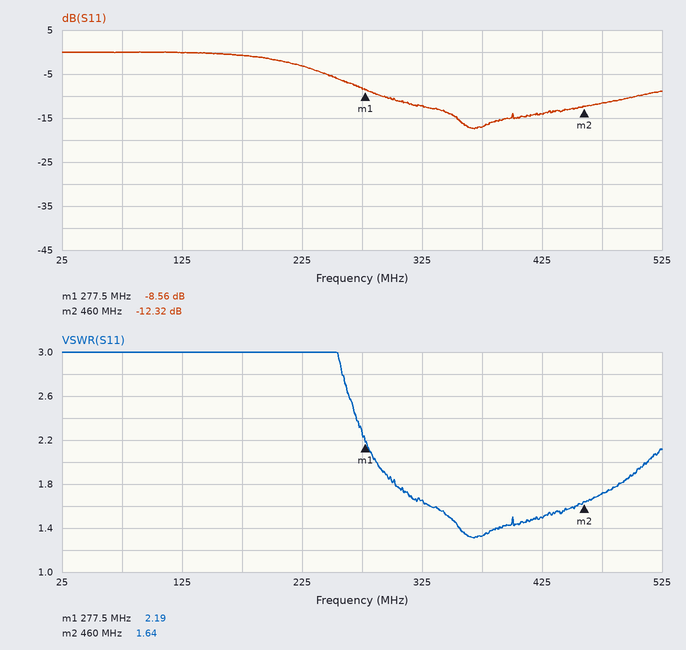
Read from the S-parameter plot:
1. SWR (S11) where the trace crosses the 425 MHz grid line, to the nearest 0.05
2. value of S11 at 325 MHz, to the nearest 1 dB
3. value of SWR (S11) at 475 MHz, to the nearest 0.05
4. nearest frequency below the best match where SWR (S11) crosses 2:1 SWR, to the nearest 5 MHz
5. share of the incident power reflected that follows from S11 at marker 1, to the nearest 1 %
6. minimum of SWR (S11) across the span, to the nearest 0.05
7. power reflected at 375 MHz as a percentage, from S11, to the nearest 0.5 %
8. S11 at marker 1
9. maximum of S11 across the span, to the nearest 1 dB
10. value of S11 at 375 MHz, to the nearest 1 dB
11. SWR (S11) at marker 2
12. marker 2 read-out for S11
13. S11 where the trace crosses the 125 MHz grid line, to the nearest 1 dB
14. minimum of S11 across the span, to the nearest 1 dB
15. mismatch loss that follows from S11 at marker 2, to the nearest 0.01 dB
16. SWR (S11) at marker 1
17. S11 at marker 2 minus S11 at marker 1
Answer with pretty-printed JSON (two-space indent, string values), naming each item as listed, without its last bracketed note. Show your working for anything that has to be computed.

{
  "SWR (S11) where the trace crosses the 425 MHz grid line, to the nearest 0.05": "1.50",
  "value of S11 at 325 MHz, to the nearest 1 dB": "-12 dB",
  "value of SWR (S11) at 475 MHz, to the nearest 0.05": "1.70",
  "nearest frequency below the best match where SWR (S11) crosses 2:1 SWR, to the nearest 5 MHz": "285 MHz",
  "share of the incident power reflected that follows from S11 at marker 1, to the nearest 1 %": "10^(-8.56/10) ≈ 14 %",
  "minimum of SWR (S11) across the span, to the nearest 0.05": "1.30",
  "power reflected at 375 MHz as a percentage, from S11, to the nearest 0.5 %": "10^(-17/10) ≈ 2.0 %",
  "S11 at marker 1": "-8.56 dB",
  "maximum of S11 across the span, to the nearest 1 dB": "0 dB",
  "value of S11 at 375 MHz, to the nearest 1 dB": "-17 dB",
  "SWR (S11) at marker 2": "1.64",
  "marker 2 read-out for S11": "-12.32 dB",
  "S11 where the trace crosses the 125 MHz grid line, to the nearest 1 dB": "0 dB",
  "minimum of S11 across the span, to the nearest 1 dB": "-17 dB",
  "mismatch loss that follows from S11 at marker 2, to the nearest 0.01 dB": "−10 log10(1 − 10^(-12.32/10)) ≈ 0.26 dB",
  "SWR (S11) at marker 1": "2.19",
  "S11 at marker 2 minus S11 at marker 1": "-12.32 − (-8.56) = -3.76 dB"
}
